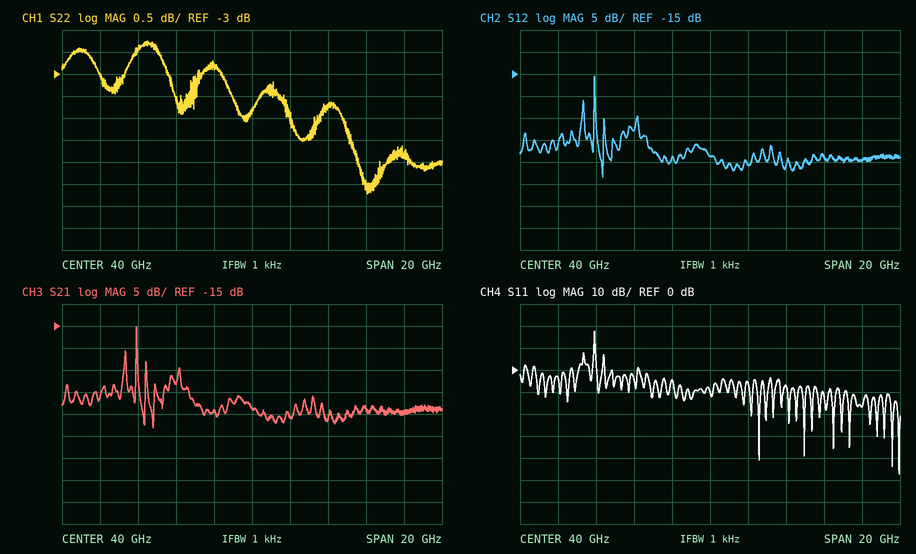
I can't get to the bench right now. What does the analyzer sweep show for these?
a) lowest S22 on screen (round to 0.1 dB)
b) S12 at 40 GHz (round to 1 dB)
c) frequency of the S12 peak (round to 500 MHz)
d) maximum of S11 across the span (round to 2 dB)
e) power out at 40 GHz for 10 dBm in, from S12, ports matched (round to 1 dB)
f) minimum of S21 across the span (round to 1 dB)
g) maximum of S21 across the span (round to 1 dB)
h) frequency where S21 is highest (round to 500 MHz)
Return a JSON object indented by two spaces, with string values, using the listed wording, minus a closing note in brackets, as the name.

{
  "lowest S22 on screen": "-5.7 dB",
  "S12 at 40 GHz": "-34 dB",
  "frequency of the S12 peak": "34.0 GHz",
  "maximum of S11 across the span": "18 dB",
  "power out at 40 GHz for 10 dBm in, from S12, ports matched": "-24 dBm",
  "minimum of S21 across the span": "-38 dB",
  "maximum of S21 across the span": "-15 dB",
  "frequency where S21 is highest": "34.0 GHz"
}
